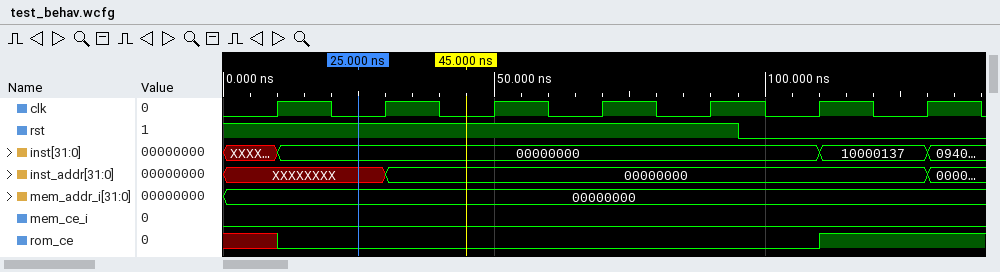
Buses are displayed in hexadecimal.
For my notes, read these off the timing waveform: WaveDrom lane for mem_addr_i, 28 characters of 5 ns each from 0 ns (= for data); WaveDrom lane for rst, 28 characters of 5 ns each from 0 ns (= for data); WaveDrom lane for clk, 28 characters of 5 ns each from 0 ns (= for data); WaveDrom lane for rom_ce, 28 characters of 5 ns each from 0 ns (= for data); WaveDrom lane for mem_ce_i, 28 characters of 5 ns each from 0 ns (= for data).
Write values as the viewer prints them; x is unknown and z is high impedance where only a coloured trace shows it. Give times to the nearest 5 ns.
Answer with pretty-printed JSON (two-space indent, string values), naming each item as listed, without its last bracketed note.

{
  "WaveDrom lane for mem_addr_i, 28 characters of 5 ns each from 0 ns": "{name: 'mem_addr_i', wave: '=...........................', data: '00000000'}",
  "WaveDrom lane for rst, 28 characters of 5 ns each from 0 ns": "{name: 'rst', wave: '1..................0........'}",
  "WaveDrom lane for clk, 28 characters of 5 ns each from 0 ns": "{name: 'clk', wave: '0.1.0.1.0.1.0.1.0.1.0.1.0.1.'}",
  "WaveDrom lane for rom_ce, 28 characters of 5 ns each from 0 ns": "{name: 'rom_ce', wave: 'x.0...................1.....'}",
  "WaveDrom lane for mem_ce_i, 28 characters of 5 ns each from 0 ns": "{name: 'mem_ce_i', wave: '0...........................'}"
}
